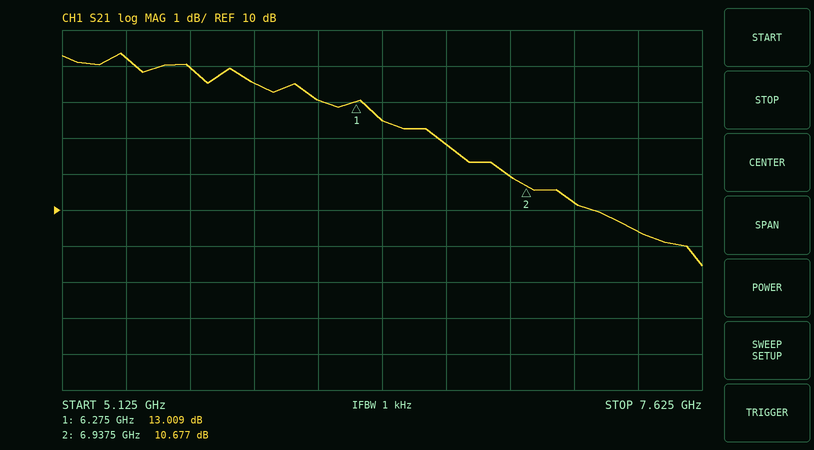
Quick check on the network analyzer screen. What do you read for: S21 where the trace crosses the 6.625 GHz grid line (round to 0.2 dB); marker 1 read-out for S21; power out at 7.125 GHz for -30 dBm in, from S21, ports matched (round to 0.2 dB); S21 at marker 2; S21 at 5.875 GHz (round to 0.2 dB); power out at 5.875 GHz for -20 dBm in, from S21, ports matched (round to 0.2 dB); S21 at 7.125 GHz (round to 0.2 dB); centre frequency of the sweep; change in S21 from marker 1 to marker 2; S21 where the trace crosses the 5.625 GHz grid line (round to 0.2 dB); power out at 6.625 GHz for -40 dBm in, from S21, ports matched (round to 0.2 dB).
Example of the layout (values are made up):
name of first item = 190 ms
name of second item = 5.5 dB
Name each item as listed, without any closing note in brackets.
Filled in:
S21 where the trace crosses the 6.625 GHz grid line = 11.8 dB
marker 1 read-out for S21 = 13.009 dB
power out at 7.125 GHz for -30 dBm in, from S21, ports matched = -19.8 dBm
S21 at marker 2 = 10.677 dB
S21 at 5.875 GHz = 13.6 dB
power out at 5.875 GHz for -20 dBm in, from S21, ports matched = -6.4 dBm
S21 at 7.125 GHz = 10.2 dB
centre frequency of the sweep = 6.375 GHz
change in S21 from marker 1 to marker 2 = -2.332 dB
S21 where the trace crosses the 5.625 GHz grid line = 14.0 dB
power out at 6.625 GHz for -40 dBm in, from S21, ports matched = -28.2 dBm
